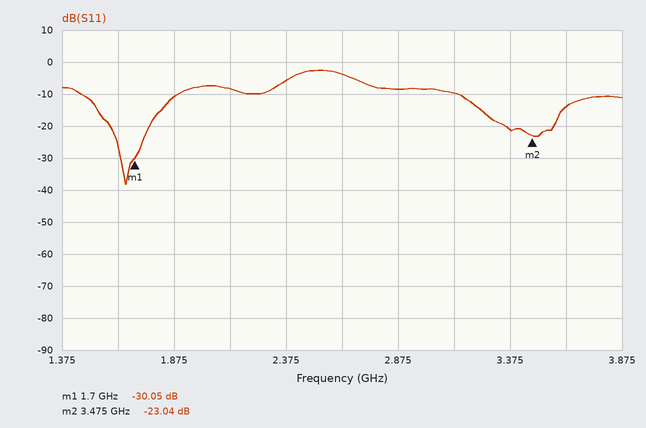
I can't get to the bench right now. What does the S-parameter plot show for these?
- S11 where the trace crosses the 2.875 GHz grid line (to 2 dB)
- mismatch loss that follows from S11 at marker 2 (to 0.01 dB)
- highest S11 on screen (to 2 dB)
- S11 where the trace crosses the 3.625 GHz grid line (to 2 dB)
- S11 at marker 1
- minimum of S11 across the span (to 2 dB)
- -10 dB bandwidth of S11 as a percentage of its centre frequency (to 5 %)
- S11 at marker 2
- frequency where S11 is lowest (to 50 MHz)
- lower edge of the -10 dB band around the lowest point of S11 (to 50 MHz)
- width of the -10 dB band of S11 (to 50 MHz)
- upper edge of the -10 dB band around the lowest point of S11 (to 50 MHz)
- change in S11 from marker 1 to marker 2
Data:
-8 dB
0.02 dB
-2 dB
-14 dB
-30.05 dB
-38 dB
25 %
-23.04 dB
1.65 GHz
1.45 GHz
450 MHz
1.90 GHz
7.01 dB
